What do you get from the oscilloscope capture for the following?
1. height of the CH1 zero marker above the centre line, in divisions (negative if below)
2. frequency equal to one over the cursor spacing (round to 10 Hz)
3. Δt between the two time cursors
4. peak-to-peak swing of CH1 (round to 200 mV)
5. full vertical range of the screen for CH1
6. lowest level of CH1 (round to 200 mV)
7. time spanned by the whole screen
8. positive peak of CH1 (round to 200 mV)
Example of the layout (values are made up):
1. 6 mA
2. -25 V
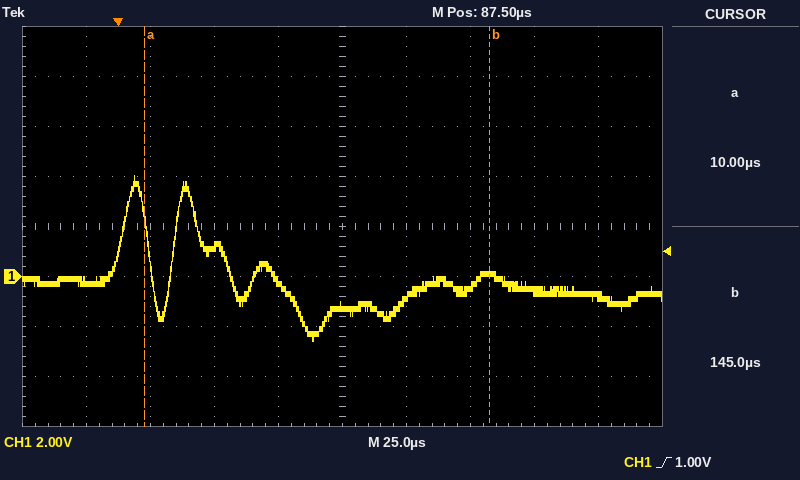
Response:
1. -1.0 div
2. 7.41 kHz
3. 135.0 µs
4. 6.6 V
5. 16 V
6. -2.6 V
7. 250 µs
8. 4.0 V
